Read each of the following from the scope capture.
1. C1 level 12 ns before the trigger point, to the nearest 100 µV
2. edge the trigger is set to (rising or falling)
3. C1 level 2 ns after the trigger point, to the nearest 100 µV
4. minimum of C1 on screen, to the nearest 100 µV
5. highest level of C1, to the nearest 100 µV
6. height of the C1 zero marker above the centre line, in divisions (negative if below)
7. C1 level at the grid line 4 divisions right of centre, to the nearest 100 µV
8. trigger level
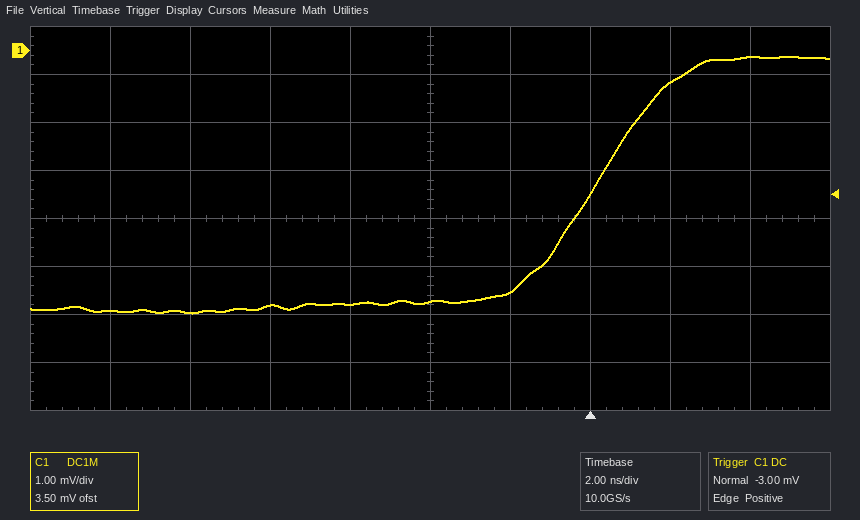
-5.4 mV
rising
-700 µV
-5.5 mV
-100 µV
+3.5 div
-100 µV
-3.00 mV
